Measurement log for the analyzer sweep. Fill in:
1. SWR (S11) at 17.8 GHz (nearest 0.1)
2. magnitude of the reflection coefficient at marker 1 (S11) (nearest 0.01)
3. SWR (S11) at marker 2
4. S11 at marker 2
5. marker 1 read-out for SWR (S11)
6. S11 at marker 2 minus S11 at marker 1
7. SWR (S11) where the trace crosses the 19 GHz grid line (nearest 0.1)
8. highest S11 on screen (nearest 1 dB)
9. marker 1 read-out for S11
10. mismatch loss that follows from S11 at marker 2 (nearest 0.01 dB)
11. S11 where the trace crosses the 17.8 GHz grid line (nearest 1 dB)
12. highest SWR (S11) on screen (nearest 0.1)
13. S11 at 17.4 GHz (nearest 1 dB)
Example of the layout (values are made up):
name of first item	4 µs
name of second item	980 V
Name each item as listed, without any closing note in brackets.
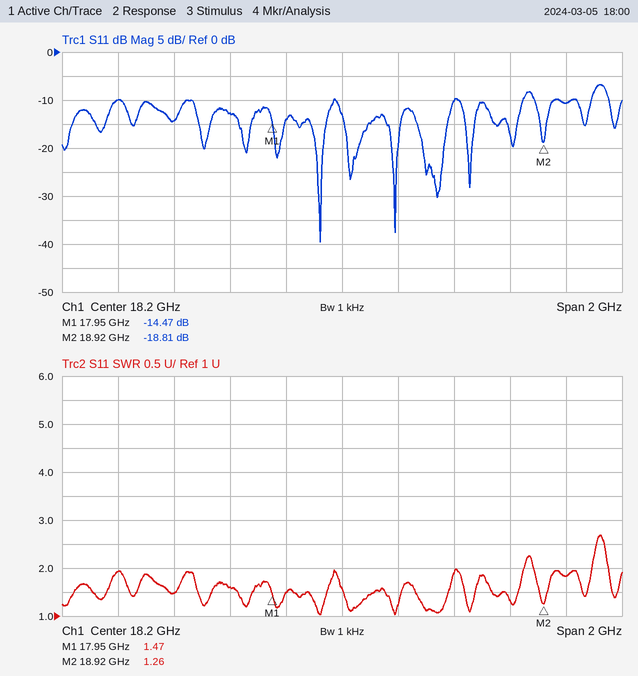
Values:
SWR (S11) at 17.8 GHz	1.6
magnitude of the reflection coefficient at marker 1 (S11)	0.19
SWR (S11) at marker 2	1.26
S11 at marker 2	-18.81 dB
marker 1 read-out for SWR	1.47
S11 at marker 2 minus S11 at marker 1	-4.34 dB
SWR (S11) where the trace crosses the 19 GHz grid line	1.8
highest S11 on screen	-7 dB
marker 1 read-out for S11	-14.47 dB
mismatch loss that follows from S11 at marker 2	0.06 dB
S11 where the trace crosses the 17.8 GHz grid line	-13 dB
highest SWR (S11) on screen	2.7
S11 at 17.4 GHz	-10 dB
